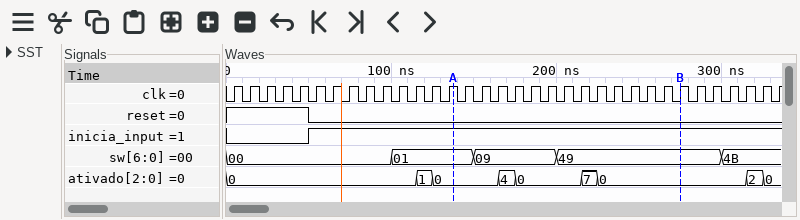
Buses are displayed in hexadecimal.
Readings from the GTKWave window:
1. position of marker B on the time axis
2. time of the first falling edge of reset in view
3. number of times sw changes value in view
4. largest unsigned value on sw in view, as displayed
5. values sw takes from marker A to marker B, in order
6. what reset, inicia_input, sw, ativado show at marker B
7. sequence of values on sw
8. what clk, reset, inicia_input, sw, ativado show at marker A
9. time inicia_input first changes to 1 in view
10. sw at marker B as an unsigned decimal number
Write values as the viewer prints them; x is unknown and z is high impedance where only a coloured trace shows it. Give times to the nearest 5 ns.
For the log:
275 ns
50 ns
4
4B
01, 09, 49
reset=0, inicia_input=1, sw=49, ativado=0
00, 01, 09, 49, 4B
clk=1, reset=0, inicia_input=1, sw=01, ativado=0
50 ns
73
